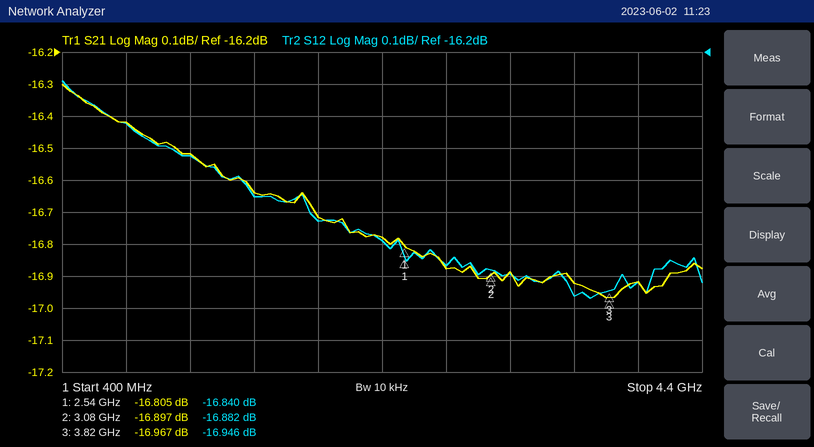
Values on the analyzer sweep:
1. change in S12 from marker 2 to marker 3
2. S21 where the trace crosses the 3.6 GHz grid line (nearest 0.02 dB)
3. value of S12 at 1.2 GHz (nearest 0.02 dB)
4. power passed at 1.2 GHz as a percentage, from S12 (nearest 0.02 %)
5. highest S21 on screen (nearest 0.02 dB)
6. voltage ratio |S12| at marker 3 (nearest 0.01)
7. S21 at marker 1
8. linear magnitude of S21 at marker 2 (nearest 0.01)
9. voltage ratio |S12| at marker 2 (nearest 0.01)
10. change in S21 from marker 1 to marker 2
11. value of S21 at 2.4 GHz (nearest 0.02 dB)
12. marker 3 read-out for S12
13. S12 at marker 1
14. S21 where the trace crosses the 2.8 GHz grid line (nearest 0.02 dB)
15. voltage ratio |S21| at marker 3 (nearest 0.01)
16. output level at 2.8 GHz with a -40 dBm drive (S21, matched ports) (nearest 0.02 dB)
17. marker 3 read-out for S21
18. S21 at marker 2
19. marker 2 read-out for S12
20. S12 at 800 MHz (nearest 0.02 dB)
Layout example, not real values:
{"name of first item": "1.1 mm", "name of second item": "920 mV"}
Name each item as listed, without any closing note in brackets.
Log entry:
{"change in S12 from marker 2 to marker 3": "-0.064 dB", "S21 where the trace crosses the 3.6 GHz grid line": "-16.92 dB", "value of S12 at 1.2 GHz": "-16.52 dB", "power passed at 1.2 GHz as a percentage, from S12": "2.22 %", "highest S21 on screen": "-16.30 dB", "voltage ratio |S12| at marker 3": "0.14", "S21 at marker 1": "-16.805 dB", "linear magnitude of S21 at marker 2": "0.14", "voltage ratio |S12| at marker 2": "0.14", "change in S21 from marker 1 to marker 2": "-0.092 dB", "value of S21 at 2.4 GHz": "-16.78 dB", "marker 3 read-out for S12": "-16.946 dB", "S12 at marker 1": "-16.840 dB", "S21 where the trace crosses the 2.8 GHz grid line": "-16.88 dB", "voltage ratio |S21| at marker 3": "0.14", "output level at 2.8 GHz with a -40 dBm drive (S21, matched ports)": "-56.88 dBm", "marker 3 read-out for S21": "-16.967 dB", "S21 at marker 2": "-16.897 dB", "marker 2 read-out for S12": "-16.882 dB", "S12 at 800 MHz": "-16.42 dB"}
